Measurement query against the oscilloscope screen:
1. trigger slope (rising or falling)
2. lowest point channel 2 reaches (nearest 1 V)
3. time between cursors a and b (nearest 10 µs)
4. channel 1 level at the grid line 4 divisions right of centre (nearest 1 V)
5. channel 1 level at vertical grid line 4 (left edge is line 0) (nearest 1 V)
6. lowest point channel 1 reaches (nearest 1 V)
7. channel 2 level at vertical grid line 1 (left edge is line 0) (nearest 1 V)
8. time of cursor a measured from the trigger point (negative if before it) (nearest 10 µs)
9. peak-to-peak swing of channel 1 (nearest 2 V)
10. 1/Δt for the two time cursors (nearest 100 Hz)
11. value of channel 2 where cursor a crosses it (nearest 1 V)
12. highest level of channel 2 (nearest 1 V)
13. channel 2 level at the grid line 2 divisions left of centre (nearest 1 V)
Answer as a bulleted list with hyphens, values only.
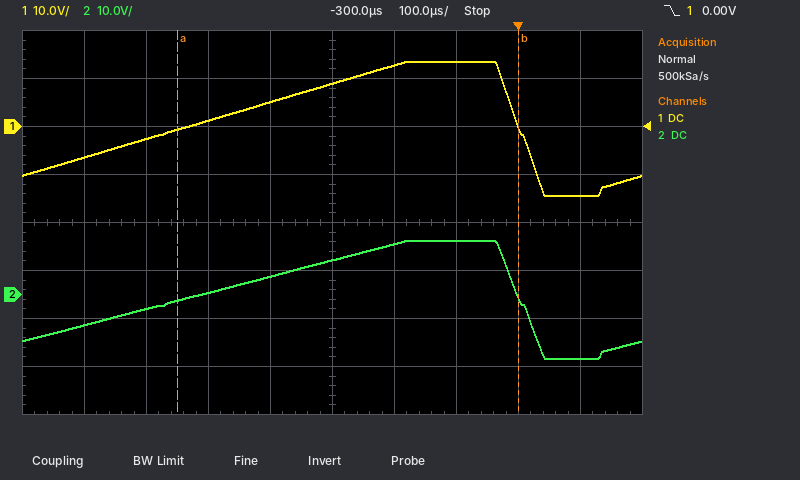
- falling
- -13 V
- 550 µs
- -14 V
- 5 V
- -14 V
- -6 V
- -550 µs
- 28 V
- 1.8 kHz
- -1 V
- 11 V
- 0 V
